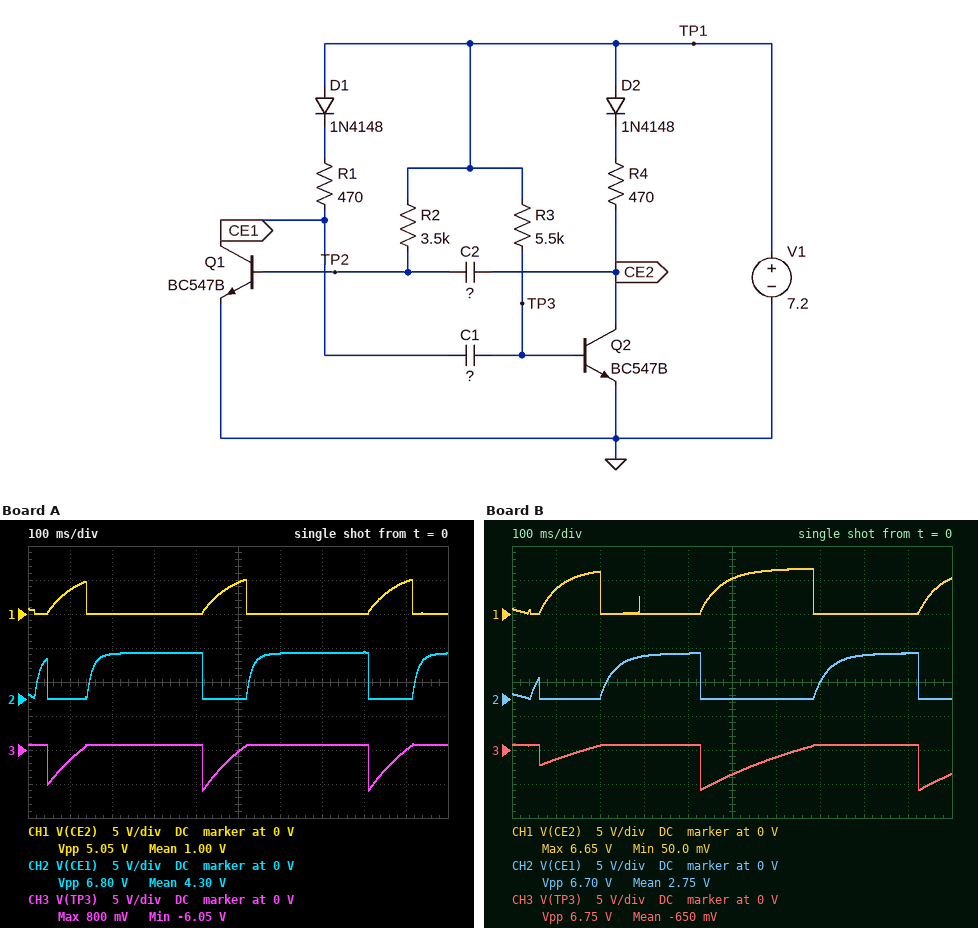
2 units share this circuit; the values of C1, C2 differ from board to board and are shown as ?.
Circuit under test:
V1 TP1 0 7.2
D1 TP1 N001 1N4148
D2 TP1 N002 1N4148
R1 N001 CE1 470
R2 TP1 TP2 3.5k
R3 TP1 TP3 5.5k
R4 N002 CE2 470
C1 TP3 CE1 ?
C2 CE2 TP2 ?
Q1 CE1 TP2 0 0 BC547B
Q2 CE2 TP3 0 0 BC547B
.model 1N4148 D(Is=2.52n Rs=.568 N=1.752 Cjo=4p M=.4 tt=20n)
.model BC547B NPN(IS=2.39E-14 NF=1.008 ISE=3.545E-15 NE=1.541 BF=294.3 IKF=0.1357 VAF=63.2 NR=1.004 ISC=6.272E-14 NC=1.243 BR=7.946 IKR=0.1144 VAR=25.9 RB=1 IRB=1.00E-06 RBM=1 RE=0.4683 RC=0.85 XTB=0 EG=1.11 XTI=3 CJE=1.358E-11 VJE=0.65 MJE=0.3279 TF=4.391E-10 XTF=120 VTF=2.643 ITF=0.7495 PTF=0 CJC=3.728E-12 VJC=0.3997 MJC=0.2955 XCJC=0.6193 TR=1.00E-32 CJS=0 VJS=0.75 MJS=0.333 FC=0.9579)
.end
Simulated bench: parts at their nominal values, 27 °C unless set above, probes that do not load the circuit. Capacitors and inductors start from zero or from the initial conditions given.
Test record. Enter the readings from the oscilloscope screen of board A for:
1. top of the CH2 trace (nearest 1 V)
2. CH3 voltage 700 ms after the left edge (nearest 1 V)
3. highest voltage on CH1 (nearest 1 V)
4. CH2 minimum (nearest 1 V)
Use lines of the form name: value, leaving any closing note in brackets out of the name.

top of the CH2 trace: 7 V
CH3 voltage 700 ms after the left edge: 1 V
highest voltage on CH1: 5 V
CH2 minimum: 0 V
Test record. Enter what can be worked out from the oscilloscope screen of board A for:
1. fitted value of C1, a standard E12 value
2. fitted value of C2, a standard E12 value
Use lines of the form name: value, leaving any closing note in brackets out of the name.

fitted value of C1, a standard E12 value: 27 µF
fitted value of C2, a standard E12 value: 150 µF
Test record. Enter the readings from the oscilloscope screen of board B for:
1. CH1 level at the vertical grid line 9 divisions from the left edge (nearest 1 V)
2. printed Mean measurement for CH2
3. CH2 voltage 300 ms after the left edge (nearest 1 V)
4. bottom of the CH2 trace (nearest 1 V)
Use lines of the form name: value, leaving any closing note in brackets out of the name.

CH1 level at the vertical grid line 9 divisions from the left edge: 0 V
printed Mean measurement for CH2: 2.75 V
CH2 voltage 300 ms after the left edge: 6 V
bottom of the CH2 trace: 0 V
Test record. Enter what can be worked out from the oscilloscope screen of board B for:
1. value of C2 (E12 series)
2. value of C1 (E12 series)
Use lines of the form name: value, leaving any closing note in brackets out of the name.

value of C2: 100 µF
value of C1: 68 µF
